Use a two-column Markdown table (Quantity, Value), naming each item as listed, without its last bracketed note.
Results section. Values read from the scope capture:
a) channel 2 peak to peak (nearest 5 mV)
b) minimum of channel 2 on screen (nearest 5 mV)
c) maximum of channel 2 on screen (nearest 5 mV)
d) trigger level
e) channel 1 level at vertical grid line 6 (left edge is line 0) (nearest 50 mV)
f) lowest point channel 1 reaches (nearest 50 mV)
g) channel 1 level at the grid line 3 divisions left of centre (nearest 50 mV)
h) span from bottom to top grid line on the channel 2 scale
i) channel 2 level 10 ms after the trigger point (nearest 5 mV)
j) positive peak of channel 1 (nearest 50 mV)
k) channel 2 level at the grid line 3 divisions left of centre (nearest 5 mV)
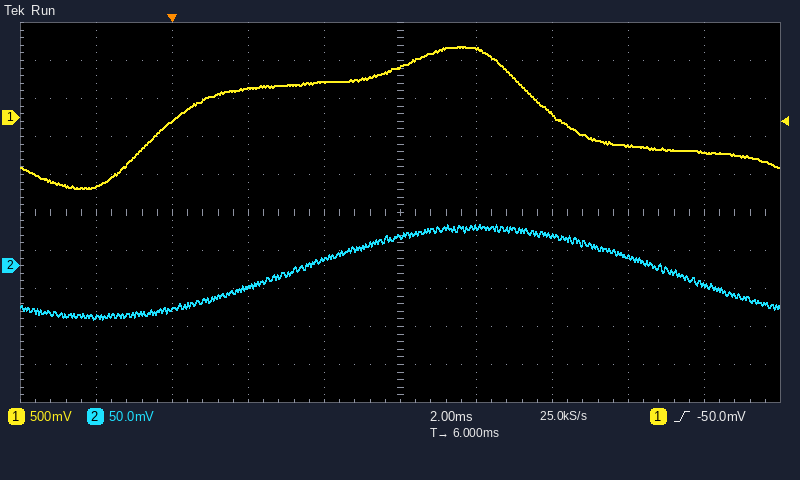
| Quantity | Value |
|---|---|
| channel 2 peak to peak | 125 mV |
| minimum of channel 2 on screen | -70 mV |
| maximum of channel 2 on screen | 55 mV |
| trigger level | -50.0 mV |
| channel 1 level at vertical grid line 6 (left edge is line 0) | 900 mV |
| lowest point channel 1 reaches | -950 mV |
| channel 1 level at the grid line 3 divisions left of centre | -50 mV |
| span from bottom to top grid line on the channel 2 scale | 500 mV |
| channel 2 level 10 ms after the trigger point | 40 mV |
| positive peak of channel 1 | 950 mV |
| channel 2 level at the grid line 3 divisions left of centre | -55 mV |
